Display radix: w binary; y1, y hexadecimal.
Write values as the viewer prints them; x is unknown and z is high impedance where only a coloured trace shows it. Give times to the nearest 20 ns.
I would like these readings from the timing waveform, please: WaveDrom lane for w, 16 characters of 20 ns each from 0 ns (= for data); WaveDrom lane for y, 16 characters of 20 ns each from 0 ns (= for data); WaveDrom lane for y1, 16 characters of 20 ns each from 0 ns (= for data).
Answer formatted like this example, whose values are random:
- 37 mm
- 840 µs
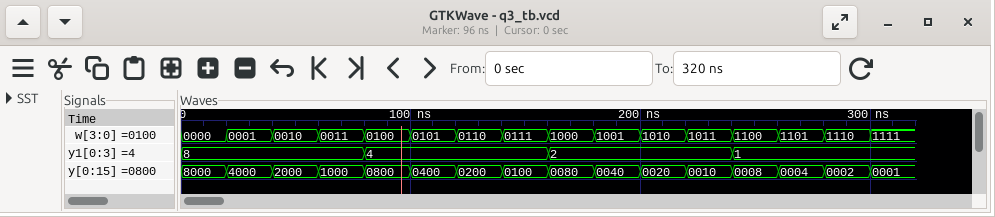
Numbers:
- {name: 'w', wave: '================', data: '0000 0001 0010 0011 0100 0101 0110 0111 1000 1001 1010 1011 1100 1101 1110 1111'}
- {name: 'y', wave: '================', data: '8000 4000 2000 1000 0800 0400 0200 0100 0080 0040 0020 0010 0008 0004 0002 0001'}
- {name: 'y1', wave: '=...=...=...=...', data: '8 4 2 1'}
